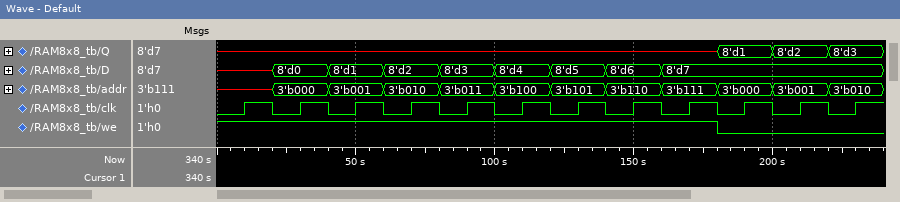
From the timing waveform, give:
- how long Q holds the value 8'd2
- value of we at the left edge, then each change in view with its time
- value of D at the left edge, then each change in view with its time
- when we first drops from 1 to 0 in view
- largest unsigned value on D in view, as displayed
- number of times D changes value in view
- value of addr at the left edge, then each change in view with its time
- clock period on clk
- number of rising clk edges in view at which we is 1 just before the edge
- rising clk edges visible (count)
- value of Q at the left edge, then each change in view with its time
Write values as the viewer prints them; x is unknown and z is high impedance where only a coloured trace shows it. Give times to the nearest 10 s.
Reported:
20 s
1, 0 at 180 s
x, 8'd0 at 20 s, 8'd1 at 40 s, 8'd2 at 60 s, 8'd3 at 80 s, 8'd4 at 100 s, 8'd5 at 120 s, 8'd6 at 140 s, 8'd7 at 160 s
180 s
8'd7
8
x, 3'b000 at 20 s, 3'b001 at 40 s, 3'b010 at 60 s, 3'b011 at 80 s, 3'b100 at 100 s, 3'b101 at 120 s, 3'b110 at 140 s, 3'b111 at 160 s, 3'b000 at 180 s, 3'b001 at 200 s, 3'b010 at 220 s
20 s
9
12
x, 8'd1 at 180 s, 8'd2 at 200 s, 8'd3 at 220 s
